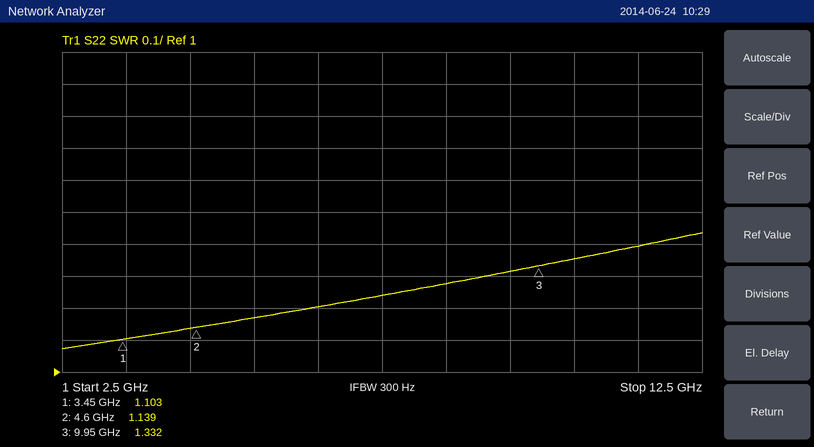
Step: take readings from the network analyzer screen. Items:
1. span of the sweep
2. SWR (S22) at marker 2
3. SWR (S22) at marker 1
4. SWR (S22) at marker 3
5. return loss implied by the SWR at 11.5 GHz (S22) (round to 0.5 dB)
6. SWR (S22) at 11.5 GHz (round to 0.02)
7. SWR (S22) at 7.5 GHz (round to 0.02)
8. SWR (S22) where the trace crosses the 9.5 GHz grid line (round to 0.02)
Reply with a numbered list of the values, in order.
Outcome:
1. 10 GHz
2. 1.139
3. 1.103
4. 1.332
5. 15.5 dB
6. 1.40
7. 1.24
8. 1.32
